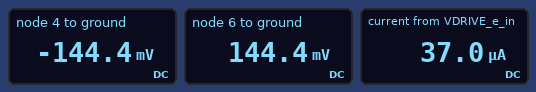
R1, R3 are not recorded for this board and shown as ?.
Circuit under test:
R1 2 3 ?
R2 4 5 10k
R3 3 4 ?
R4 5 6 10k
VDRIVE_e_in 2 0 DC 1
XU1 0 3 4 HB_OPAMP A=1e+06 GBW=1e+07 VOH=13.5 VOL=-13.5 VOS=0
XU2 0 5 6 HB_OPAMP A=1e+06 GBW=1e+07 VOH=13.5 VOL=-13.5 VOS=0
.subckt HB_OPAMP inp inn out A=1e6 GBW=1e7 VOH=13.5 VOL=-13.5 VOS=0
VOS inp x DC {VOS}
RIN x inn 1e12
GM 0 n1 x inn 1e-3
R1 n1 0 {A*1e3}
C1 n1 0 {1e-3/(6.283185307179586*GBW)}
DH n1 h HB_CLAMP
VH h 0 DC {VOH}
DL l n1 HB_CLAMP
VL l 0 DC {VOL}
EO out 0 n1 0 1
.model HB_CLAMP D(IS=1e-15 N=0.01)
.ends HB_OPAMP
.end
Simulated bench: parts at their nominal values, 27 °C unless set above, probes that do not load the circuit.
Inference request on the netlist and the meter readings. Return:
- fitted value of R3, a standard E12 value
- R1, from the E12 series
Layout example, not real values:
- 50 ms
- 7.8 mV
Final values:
- 3.9 kΩ
- 27 kΩ
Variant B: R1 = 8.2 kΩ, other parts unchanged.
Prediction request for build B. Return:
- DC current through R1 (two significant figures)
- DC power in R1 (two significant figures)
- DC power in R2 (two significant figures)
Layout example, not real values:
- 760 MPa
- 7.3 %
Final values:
- 120 µA
- 120 µW
- 23 µW
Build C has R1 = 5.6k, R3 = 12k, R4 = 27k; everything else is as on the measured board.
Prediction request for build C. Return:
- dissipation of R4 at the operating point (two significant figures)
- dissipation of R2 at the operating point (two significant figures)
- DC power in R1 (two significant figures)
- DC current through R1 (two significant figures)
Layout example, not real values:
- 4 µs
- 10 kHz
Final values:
- 1.2 mW
- 460 µW
- 180 µW
- 180 µA
